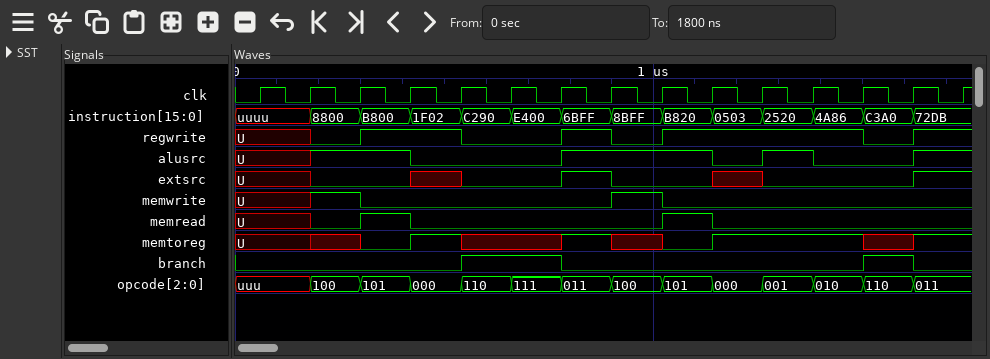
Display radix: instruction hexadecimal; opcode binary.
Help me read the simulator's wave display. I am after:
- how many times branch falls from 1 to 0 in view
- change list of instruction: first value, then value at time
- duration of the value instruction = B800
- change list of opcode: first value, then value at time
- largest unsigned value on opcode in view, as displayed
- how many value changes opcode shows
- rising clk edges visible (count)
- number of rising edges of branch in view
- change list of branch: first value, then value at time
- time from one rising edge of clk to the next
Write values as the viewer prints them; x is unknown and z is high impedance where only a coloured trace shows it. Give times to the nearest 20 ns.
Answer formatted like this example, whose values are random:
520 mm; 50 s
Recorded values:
2; uuuu, 8800 at 180 ns, B800 at 300 ns, 1F02 at 420 ns, C290 at 540 ns, E400 at 660 ns, 6BFF at 780 ns, 8BFF at 900 ns, B820 at 1020 ns, 0503 at 1140 ns, 2520 at 1260 ns, 4A86 at 1380 ns, C3A0 at 1500 ns, 72DB at 1620 ns; 120 ns; uuu, 100 at 180 ns, 101 at 300 ns, 000 at 420 ns, 110 at 540 ns, 111 at 660 ns, 011 at 780 ns, 100 at 900 ns, 101 at 1020 ns, 000 at 1140 ns, 001 at 1260 ns, 010 at 1380 ns, 110 at 1500 ns, 011 at 1620 ns; 111; 13; 15; 2; 0, 1 at 540 ns, 0 at 780 ns, 1 at 1500 ns, 0 at 1620 ns; 120 ns
